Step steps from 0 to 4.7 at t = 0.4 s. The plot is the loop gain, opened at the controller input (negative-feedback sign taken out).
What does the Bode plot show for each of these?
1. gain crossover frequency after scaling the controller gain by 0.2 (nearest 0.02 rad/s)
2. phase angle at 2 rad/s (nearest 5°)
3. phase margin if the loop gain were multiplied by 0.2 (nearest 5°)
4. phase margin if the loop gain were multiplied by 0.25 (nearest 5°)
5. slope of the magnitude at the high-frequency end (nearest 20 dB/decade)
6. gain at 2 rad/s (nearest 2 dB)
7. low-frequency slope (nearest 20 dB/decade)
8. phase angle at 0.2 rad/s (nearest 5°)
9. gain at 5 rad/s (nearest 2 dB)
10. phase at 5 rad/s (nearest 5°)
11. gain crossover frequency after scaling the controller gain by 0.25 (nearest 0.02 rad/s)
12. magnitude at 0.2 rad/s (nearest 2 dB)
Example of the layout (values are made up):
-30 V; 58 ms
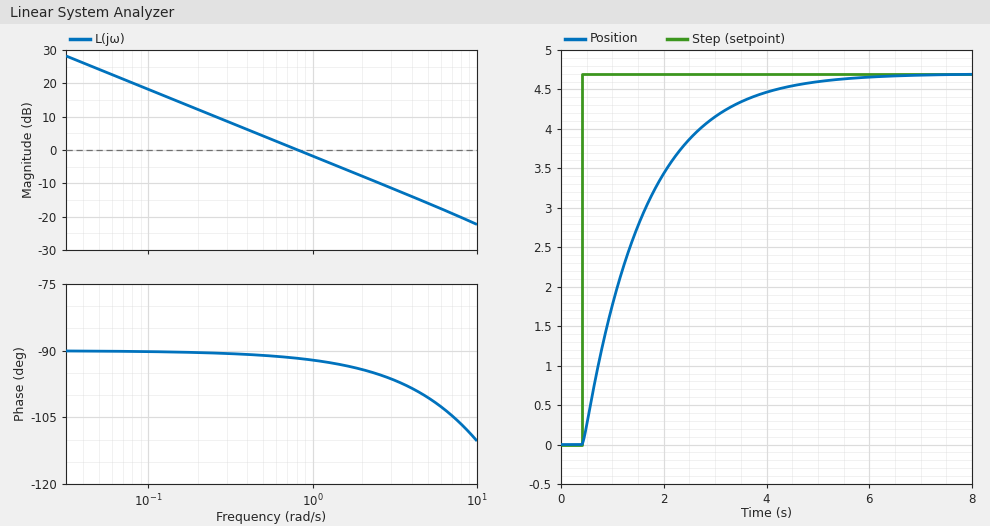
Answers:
0.16 rad/s; -95°; 90°; 90°; -20 dB/decade; -8 dB; -20 dB/decade; -90°; -16 dB; -100°; 0.20 rad/s; 12 dB
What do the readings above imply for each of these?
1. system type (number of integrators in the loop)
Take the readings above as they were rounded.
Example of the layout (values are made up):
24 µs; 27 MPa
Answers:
1
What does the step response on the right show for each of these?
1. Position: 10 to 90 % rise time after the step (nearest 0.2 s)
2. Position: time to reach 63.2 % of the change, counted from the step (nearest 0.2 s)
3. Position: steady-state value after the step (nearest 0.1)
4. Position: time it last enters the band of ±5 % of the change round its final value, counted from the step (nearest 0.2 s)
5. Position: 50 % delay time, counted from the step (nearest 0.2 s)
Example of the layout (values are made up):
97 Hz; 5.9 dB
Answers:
2.6 s; 1.2 s; 4.7; 3.6 s; 0.8 s
